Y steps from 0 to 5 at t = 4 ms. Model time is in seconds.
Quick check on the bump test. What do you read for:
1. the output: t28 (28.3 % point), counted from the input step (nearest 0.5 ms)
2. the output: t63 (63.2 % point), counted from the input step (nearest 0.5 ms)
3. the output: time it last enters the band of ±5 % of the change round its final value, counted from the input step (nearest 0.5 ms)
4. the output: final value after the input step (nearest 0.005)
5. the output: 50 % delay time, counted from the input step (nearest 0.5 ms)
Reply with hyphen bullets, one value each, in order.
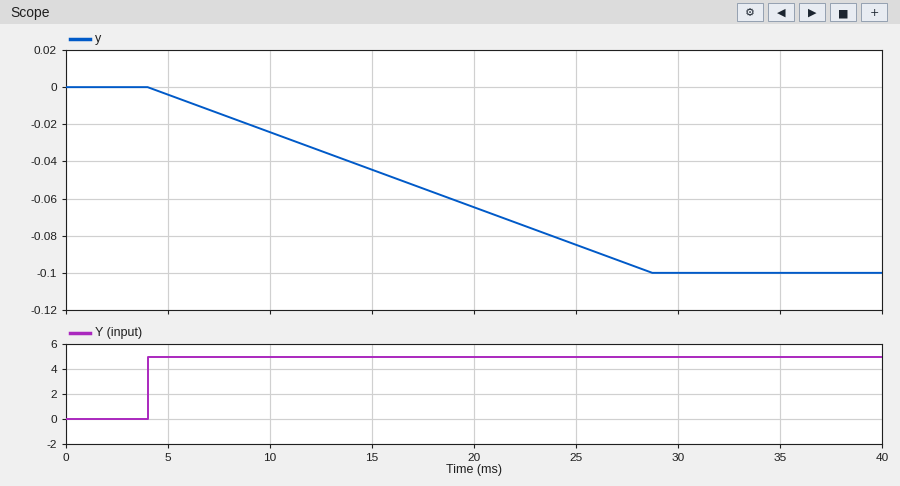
- 7.0 ms
- 15.5 ms
- 23.5 ms
- -0.100
- 12.5 ms
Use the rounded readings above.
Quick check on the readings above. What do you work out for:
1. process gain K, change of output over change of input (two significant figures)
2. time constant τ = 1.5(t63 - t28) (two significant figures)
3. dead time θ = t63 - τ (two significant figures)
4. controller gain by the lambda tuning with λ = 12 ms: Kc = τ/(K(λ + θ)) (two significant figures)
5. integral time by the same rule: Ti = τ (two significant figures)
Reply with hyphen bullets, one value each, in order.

- -0.020
- 13 ms
- 2.5 ms
- -45
- 13 ms
